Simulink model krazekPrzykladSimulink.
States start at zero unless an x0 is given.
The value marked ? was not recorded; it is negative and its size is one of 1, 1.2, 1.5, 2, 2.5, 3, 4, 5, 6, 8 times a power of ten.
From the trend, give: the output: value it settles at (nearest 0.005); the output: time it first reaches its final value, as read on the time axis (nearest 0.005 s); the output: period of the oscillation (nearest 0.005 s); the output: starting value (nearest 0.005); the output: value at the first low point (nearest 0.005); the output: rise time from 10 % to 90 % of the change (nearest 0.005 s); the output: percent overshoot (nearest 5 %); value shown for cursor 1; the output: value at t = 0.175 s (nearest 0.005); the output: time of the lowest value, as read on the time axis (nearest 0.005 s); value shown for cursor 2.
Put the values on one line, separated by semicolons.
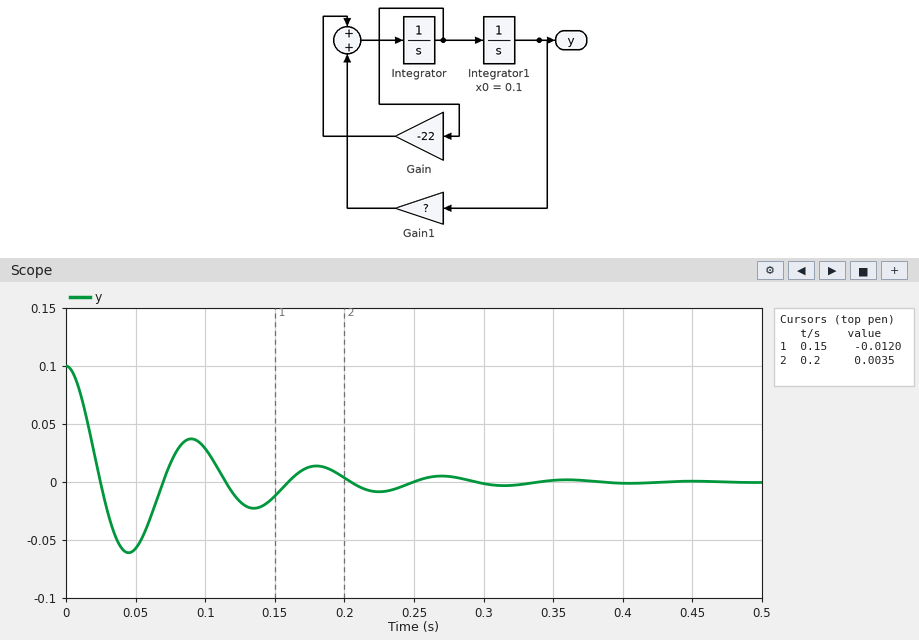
0.000; 0.025 s; 0.090 s; 0.100; -0.060; 0.015 s; 60 %; -0.0120; 0.015; 0.045 s; 0.0035
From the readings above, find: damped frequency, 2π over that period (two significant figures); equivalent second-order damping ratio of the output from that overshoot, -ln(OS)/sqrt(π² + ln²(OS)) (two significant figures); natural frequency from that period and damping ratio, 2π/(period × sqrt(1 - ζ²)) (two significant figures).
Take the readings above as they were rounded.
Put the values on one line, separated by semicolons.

70 rad/s; 0.16; 71 rad/s
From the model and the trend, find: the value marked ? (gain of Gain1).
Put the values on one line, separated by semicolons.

-5000
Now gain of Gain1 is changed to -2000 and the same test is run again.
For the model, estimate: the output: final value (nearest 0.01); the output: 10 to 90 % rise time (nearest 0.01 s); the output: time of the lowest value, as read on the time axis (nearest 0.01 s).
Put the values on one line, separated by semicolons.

0.00; 0.03 s; 0.07 s
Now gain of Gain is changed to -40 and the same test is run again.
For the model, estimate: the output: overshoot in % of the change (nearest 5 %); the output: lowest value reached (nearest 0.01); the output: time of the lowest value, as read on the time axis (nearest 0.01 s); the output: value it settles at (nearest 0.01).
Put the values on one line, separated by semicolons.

40 %; -0.04; 0.05 s; 0.00
